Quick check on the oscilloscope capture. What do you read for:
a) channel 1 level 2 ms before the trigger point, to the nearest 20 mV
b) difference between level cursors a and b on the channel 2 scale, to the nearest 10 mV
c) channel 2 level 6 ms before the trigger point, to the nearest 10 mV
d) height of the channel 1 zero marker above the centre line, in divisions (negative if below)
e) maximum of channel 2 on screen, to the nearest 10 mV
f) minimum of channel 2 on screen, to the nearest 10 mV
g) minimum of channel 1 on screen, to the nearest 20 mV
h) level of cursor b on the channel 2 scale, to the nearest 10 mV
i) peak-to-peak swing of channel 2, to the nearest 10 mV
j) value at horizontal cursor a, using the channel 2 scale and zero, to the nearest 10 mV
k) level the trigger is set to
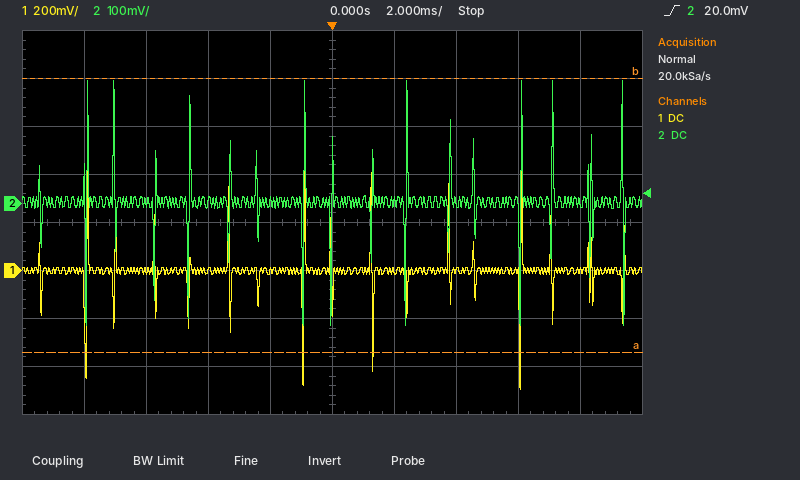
0 mV
570 mV
0 mV
-1.0 div
260 mV
-250 mV
-500 mV
260 mV
510 mV
-310 mV
20.0 mV
